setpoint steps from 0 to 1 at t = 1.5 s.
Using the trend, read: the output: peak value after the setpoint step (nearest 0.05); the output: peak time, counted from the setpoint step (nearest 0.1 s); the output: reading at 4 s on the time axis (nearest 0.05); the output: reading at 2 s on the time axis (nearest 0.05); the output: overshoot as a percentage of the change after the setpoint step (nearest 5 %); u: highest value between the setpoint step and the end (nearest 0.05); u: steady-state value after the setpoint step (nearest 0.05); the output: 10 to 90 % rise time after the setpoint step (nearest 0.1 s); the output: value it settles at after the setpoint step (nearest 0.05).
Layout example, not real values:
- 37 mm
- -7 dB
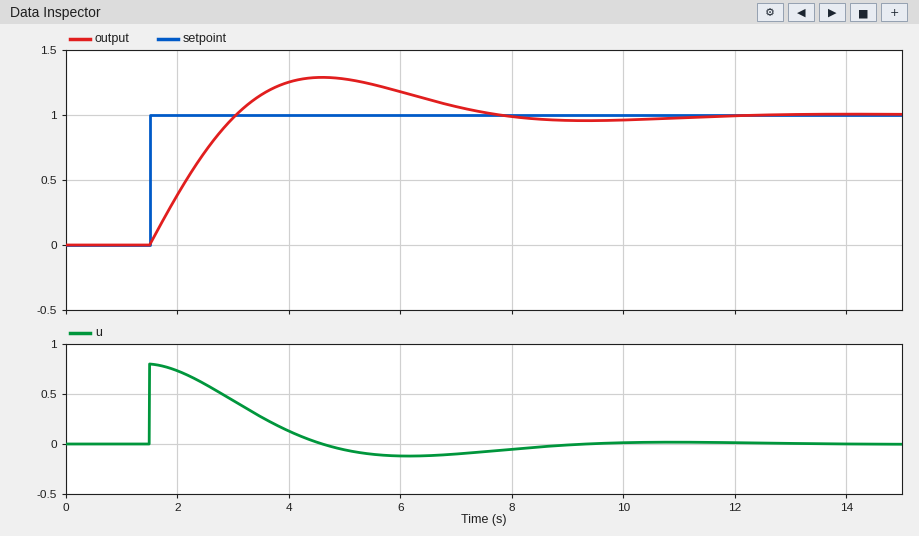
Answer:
- 1.30
- 3.1 s
- 1.25
- 0.40
- 30 %
- 0.80
- 0.00
- 1.2 s
- 1.00
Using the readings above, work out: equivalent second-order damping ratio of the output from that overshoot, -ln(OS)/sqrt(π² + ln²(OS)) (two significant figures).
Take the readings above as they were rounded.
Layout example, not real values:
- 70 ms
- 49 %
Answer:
- 0.36
